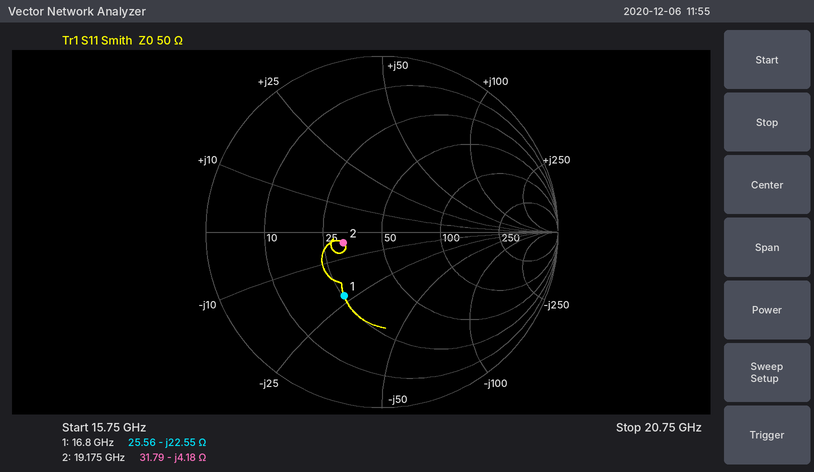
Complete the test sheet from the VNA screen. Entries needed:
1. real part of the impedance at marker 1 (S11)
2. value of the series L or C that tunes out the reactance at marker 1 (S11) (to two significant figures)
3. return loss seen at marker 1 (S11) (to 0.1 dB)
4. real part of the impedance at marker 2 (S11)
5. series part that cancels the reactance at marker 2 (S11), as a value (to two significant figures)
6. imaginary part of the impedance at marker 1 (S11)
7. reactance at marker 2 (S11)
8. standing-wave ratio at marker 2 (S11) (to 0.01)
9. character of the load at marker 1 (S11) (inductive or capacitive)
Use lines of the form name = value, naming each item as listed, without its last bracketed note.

real part of the impedance at marker 1 = 25.56 Ω
value of the series L or C that tunes out the reactance at marker 1 (S11) = 210 pH
return loss seen at marker 1 (S11) = 7.5 dB
real part of the impedance at marker 2 = 31.79 Ω
series part that cancels the reactance at marker 2 (S11), as a value = 35 pH
imaginary part of the impedance at marker 1 = -22.55 Ω
reactance at marker 2 = -4.18 Ω
standing-wave ratio at marker 2 (S11) = 1.59
character of the load at marker 1 (S11) = capacitive
